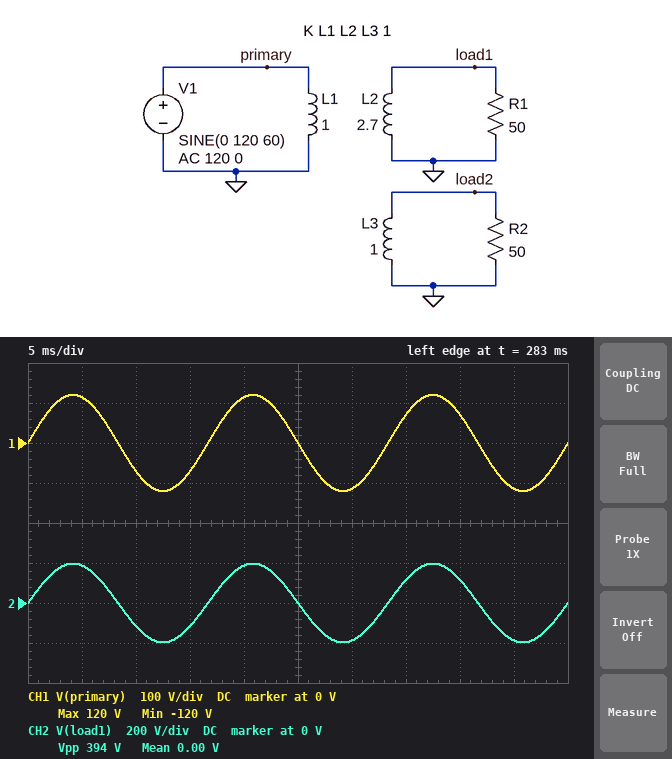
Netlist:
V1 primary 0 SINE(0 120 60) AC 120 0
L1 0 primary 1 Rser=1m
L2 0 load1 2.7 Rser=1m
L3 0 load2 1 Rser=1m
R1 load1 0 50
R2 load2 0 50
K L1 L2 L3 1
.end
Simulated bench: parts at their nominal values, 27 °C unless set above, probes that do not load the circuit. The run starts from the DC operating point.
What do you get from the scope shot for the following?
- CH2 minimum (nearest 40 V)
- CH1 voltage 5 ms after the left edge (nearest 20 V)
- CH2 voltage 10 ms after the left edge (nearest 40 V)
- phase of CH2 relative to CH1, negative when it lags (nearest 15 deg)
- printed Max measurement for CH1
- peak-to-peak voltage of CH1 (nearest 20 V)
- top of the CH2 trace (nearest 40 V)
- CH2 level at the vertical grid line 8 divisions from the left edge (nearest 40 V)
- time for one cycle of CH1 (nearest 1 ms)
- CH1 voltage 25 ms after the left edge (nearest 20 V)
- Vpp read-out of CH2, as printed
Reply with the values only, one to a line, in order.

-200 V
120 V
-120 V
0 deg
120 V
240 V
200 V
120 V
17 ms
0 V
394 V
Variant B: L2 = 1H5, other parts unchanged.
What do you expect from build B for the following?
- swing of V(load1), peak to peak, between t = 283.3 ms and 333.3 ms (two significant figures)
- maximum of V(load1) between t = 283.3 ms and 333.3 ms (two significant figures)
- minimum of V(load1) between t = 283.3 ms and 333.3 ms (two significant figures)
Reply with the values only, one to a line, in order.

290 V
150 V
-150 V
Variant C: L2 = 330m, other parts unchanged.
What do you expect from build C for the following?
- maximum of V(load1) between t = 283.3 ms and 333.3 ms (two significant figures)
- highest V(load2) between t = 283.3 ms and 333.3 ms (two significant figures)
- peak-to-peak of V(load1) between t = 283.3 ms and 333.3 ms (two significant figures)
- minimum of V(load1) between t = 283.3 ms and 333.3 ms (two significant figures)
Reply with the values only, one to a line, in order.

69 V
120 V
140 V
-69 V
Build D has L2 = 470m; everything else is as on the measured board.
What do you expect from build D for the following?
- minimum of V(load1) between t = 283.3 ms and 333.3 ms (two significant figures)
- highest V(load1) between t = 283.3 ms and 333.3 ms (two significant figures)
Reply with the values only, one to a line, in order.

-82 V
82 V
